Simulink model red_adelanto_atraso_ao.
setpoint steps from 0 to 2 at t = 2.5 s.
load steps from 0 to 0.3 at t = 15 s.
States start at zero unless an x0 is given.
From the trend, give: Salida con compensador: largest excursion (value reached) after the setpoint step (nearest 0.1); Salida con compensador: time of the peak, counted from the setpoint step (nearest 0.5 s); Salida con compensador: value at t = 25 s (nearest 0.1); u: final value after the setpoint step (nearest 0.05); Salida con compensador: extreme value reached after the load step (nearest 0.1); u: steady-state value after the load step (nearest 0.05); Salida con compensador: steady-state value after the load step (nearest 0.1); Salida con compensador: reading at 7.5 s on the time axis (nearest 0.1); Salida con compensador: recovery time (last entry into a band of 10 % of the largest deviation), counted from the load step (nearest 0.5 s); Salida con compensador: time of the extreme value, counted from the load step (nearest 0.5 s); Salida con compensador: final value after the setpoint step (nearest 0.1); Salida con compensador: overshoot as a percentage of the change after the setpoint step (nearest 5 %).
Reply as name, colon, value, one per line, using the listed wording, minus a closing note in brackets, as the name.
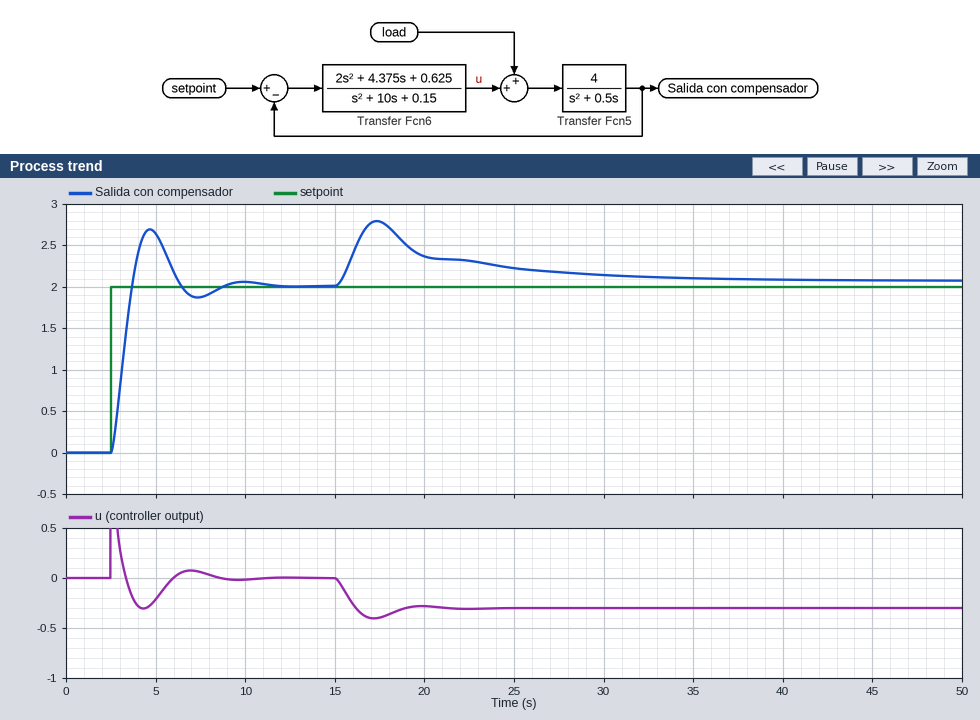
Salida con compensador: largest excursion (value reached) after the setpoint step: 2.7
Salida con compensador: time of the peak, counted from the setpoint step: 2.0 s
Salida con compensador: value at t = 25 s: 2.2
u: final value after the setpoint step: 0.00
Salida con compensador: extreme value reached after the load step: 2.8
u: steady-state value after the load step: -0.30
Salida con compensador: steady-state value after the load step: 2.1
Salida con compensador: reading at 7.5 s on the time axis: 1.9
Salida con compensador: recovery time (last entry into a band of 10 % of the largest deviation), counted from the load step: 14.5 s
Salida con compensador: time of the extreme value, counted from the load step: 2.5 s
Salida con compensador: final value after the setpoint step: 2.0
Salida con compensador: overshoot as a percentage of the change after the setpoint step: 35 %
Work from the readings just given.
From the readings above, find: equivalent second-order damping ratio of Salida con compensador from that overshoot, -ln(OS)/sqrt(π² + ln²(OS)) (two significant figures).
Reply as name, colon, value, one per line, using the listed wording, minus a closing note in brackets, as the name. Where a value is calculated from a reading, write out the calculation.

equivalent second-order damping ratio of Salida con compensador from that overshoot, -ln(OS)/sqrt(π² + ln²(OS)): ln(0.35) = -1.050; 1.050 / sqrt(9.870 + 1.102) = 0.32
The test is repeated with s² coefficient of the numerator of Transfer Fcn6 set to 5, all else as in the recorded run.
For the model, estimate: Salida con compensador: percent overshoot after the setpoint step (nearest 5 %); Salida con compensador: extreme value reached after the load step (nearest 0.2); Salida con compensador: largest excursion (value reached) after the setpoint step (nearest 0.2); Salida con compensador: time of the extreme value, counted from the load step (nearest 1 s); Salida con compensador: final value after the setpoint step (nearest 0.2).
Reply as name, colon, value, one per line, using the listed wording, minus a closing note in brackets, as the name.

Salida con compensador: percent overshoot after the setpoint step: 10 %
Salida con compensador: extreme value reached after the load step: 2.6
Salida con compensador: largest excursion (value reached) after the setpoint step: 2.2
Salida con compensador: time of the extreme value, counted from the load step: 3 s
Salida con compensador: final value after the setpoint step: 2.0
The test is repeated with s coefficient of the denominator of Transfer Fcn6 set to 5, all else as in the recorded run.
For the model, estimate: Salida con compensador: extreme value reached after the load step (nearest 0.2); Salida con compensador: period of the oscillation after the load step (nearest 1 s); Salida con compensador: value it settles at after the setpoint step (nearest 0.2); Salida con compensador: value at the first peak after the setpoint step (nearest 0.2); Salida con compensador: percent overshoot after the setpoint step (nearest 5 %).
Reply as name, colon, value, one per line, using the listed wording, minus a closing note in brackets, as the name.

Salida con compensador: extreme value reached after the load step: 2.4
Salida con compensador: period of the oscillation after the load step: 3 s
Salida con compensador: value it settles at after the setpoint step: 2.0
Salida con compensador: value at the first peak after the setpoint step: 2.8
Salida con compensador: percent overshoot after the setpoint step: 45 %
